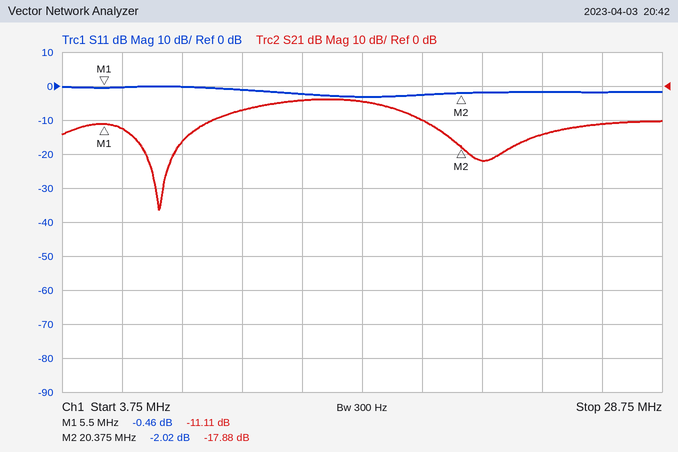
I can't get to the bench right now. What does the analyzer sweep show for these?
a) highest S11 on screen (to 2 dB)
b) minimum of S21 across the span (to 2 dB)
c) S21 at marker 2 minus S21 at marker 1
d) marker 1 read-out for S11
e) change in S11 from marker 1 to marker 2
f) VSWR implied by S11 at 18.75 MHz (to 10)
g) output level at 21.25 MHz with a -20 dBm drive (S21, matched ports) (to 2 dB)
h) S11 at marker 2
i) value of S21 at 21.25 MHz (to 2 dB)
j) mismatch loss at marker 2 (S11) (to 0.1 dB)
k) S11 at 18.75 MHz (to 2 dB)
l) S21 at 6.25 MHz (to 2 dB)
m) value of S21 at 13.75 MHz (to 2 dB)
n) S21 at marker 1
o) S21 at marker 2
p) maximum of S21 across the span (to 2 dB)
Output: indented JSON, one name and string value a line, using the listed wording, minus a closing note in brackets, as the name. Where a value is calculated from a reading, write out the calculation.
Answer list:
{
  "highest S11 on screen": "0 dB",
  "minimum of S21 across the span": "-36 dB",
  "S21 at marker 2 minus S21 at marker 1": "-17.88 − (-11.11) = -6.77 dB",
  "marker 1 read-out for S11": "-0.46 dB",
  "change in S11 from marker 1 to marker 2": "-2.02 − (-0.46) = -1.56 dB",
  "VSWR implied by S11 at 18.75 MHz": "|Γ| = 10^(-2/20) = 0.7943; VSWR = (1 + 0.7943)/(1 − 0.7943) ≈ 8.72, so 10 to the nearest 10",
  "output level at 21.25 MHz with a -20 dBm drive (S21, matched ports)": "-20 dBm + (-22 dB) = -42 dBm",
  "S11 at marker 2": "-2.02 dB",
  "value of S21 at 21.25 MHz": "-22 dB",
  "mismatch loss at marker 2 (S11)": "−10 log10(1 − 10^(-2.02/10)) ≈ 4.3 dB",
  "S11 at 18.75 MHz": "-2 dB",
  "S21 at 6.25 MHz": "-12 dB",
  "value of S21 at 13.75 MHz": "-4 dB",
  "S21 at marker 1": "-11.11 dB",
  "S21 at marker 2": "-17.88 dB",
  "maximum of S21 across the span": "-4 dB"
}
